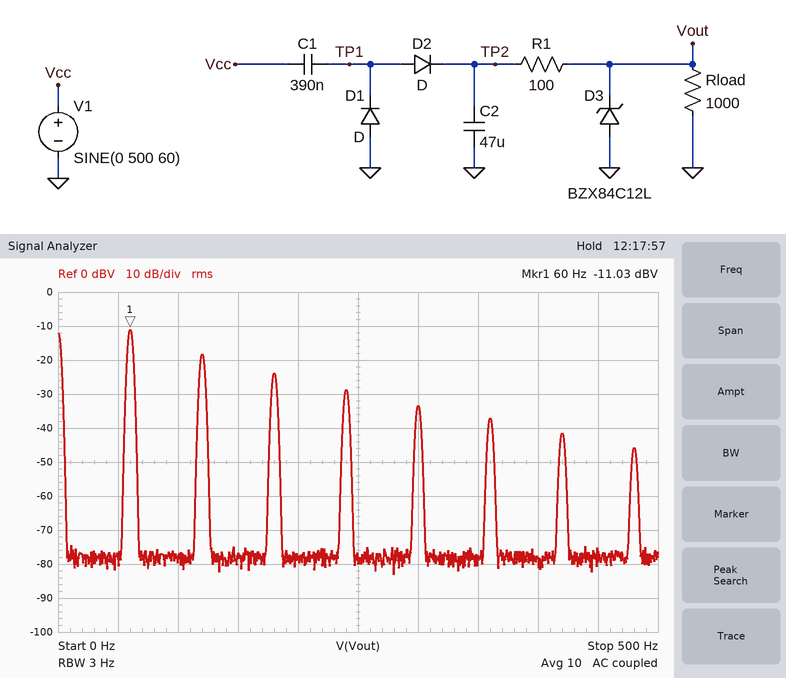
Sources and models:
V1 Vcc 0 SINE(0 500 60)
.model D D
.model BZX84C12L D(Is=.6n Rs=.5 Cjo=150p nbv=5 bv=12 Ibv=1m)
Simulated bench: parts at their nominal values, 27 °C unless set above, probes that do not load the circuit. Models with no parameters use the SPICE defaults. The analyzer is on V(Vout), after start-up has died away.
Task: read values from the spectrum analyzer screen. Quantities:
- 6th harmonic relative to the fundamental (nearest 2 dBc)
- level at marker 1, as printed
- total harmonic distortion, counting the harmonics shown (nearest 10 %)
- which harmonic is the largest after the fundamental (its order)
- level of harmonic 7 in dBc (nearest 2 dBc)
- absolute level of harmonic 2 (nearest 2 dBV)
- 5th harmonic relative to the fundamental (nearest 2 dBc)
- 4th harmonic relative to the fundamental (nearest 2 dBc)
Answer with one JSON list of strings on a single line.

["-26 dBc", "-11.03 dBV", "50 %", "2", "-30 dBc", "-18 dBV", "-22 dBc", "-18 dBc"]
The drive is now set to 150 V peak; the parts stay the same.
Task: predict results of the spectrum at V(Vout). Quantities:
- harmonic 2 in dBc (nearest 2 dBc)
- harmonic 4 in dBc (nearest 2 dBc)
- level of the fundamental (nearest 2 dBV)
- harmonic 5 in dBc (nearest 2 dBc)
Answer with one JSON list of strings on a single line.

["-12 dBc", "-32 dBc", "-8 dBV", "-44 dBc"]
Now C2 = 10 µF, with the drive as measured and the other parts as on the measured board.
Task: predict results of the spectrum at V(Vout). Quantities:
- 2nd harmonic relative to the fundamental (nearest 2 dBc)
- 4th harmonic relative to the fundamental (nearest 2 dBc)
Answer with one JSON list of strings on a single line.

["-12 dBc", "-20 dBc"]
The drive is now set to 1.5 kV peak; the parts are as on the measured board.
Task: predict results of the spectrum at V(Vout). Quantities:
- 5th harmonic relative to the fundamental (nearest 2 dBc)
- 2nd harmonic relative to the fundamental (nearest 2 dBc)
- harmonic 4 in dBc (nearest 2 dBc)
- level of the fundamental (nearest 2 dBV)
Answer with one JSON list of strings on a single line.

["-28 dBc", "-12 dBc", "-24 dBc", "-18 dBV"]
